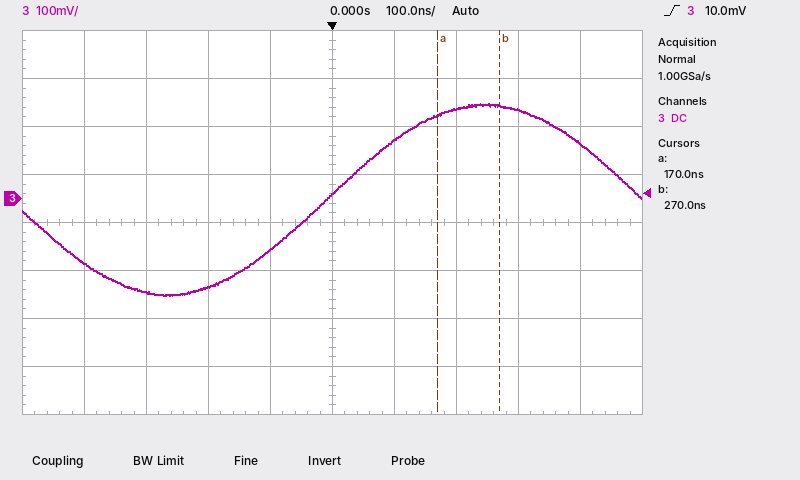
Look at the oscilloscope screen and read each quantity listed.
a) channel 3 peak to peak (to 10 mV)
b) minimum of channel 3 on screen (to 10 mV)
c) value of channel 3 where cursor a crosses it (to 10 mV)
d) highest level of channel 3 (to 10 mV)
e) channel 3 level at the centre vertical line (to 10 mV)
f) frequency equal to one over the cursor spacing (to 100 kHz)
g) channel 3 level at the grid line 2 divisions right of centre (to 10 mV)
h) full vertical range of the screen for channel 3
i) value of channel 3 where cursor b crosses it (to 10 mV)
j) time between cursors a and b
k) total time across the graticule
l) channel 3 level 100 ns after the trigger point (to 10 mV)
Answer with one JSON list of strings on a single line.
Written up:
["400 mV", "-200 mV", "170 mV", "200 mV", "10 mV", "10.0 MHz", "190 mV", "800 mV", "190 mV", "100 ns", "1 µs", "120 mV"]
